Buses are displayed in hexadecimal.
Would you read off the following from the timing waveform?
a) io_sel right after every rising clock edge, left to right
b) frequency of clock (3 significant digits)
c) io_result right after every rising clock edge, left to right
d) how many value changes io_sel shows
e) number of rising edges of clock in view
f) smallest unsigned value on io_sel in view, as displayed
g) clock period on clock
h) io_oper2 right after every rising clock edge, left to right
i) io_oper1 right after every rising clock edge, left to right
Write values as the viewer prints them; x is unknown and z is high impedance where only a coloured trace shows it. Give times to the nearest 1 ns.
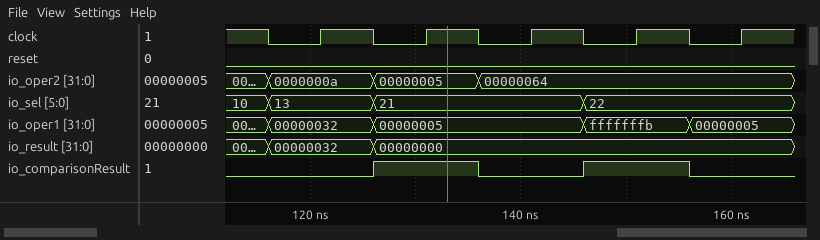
13, 21, 21, 22, 22
100 MHz
00000032, 00000000, 00000000, 00000000, 00000000
3
5
10
10 ns
0000000a, 00000005, 00000064, 00000064, 00000064
00000032, 00000005, 00000005, fffffffb, 00000005
